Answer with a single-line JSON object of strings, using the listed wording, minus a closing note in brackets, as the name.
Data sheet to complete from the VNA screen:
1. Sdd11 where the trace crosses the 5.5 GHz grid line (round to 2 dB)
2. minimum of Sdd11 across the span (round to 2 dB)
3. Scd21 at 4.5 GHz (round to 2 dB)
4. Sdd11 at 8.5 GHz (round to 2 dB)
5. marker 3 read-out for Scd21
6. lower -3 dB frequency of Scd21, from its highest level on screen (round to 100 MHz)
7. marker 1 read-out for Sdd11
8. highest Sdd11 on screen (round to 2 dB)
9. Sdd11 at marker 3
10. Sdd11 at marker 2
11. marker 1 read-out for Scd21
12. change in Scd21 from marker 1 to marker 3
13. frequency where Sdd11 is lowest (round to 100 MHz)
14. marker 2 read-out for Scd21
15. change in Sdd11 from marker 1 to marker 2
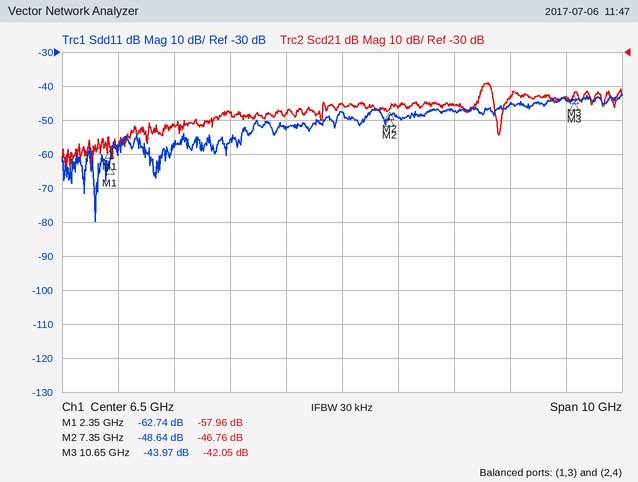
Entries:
{"Sdd11 where the trace crosses the 5.5 GHz grid line": "-52 dB", "minimum of Sdd11 across the span": "-80 dB", "Scd21 at 4.5 GHz": "-48 dB", "Sdd11 at 8.5 GHz": "-48 dB", "marker 3 read-out for Scd21": "-42.05 dB", "lower -3 dB frequency of Scd21, from its highest level on screen": "9.0 GHz", "marker 1 read-out for Sdd11": "-62.74 dB", "highest Sdd11 on screen": "-42 dB", "Sdd11 at marker 3": "-43.97 dB", "Sdd11 at marker 2": "-48.64 dB", "marker 1 read-out for Scd21": "-57.96 dB", "change in Scd21 from marker 1 to marker 3": "15.91 dB", "frequency where Sdd11 is lowest": "2.1 GHz", "marker 2 read-out for Scd21": "-46.76 dB", "change in Sdd11 from marker 1 to marker 2": "14.10 dB"}
